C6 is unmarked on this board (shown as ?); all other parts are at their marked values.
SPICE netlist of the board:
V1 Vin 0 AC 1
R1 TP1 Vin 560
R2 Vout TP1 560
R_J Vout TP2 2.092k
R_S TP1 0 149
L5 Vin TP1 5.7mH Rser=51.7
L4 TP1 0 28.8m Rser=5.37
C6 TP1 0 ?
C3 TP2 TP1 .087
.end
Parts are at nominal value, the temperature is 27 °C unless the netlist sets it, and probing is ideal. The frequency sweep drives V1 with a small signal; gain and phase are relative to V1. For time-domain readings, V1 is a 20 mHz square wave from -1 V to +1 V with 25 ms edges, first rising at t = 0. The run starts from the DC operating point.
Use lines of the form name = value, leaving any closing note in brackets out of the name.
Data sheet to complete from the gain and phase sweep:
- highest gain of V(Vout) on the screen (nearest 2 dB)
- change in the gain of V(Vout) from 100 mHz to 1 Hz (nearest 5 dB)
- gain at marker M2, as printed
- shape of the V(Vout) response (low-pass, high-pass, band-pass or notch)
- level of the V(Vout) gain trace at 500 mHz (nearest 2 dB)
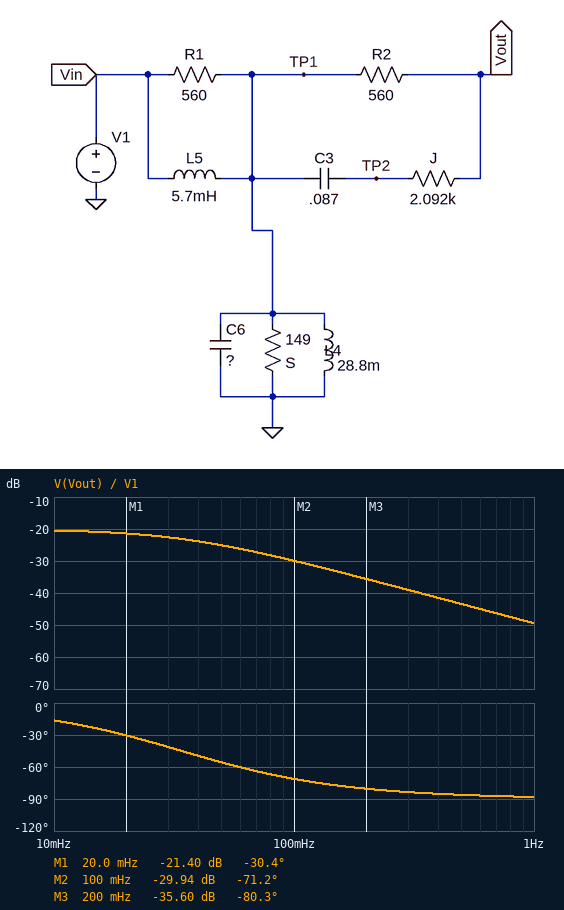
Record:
highest gain of V(Vout) on the screen = -20 dB
change in the gain of V(Vout) from 100 mHz to 1 Hz = -20 dB
gain at marker M2, as printed = -29.94 dB
shape of the V(Vout) response = low-pass
level of the V(Vout) gain trace at 500 mHz = -44 dB
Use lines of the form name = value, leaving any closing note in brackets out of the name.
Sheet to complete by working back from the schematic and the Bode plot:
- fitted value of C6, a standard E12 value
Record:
fitted value of C6, a standard E12 value = 1 F
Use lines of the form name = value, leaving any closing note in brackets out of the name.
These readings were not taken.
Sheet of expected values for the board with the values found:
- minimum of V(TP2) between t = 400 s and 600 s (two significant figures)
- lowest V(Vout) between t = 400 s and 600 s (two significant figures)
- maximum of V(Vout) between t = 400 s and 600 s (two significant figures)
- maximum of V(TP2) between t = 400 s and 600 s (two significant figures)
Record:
minimum of V(TP2) between t = 400 s and 600 s = -98 mV
lowest V(Vout) between t = 400 s and 600 s = -98 mV
maximum of V(Vout) between t = 400 s and 600 s = 98 mV
maximum of V(TP2) between t = 400 s and 600 s = 98 mV
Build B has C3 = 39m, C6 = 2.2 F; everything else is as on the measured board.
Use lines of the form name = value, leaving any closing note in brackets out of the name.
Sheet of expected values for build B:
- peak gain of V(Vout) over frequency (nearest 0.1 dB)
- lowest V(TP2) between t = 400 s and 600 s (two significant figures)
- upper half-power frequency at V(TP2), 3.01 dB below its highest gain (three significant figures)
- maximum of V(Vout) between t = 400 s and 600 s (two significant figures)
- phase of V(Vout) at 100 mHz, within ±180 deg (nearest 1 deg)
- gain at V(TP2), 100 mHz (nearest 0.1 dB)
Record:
peak gain of V(Vout) over frequency = -20.1 dB
lowest V(TP2) between t = 400 s and 600 s = -83 mV
upper half-power frequency at V(TP2), 3.01 dB below its highest gain = 15.5 mHz
maximum of V(Vout) between t = 400 s and 600 s = 83 mV
phase of V(Vout) at 100 mHz, within ±180 deg = -81 deg
gain at V(TP2), 100 mHz = -36.4 dB
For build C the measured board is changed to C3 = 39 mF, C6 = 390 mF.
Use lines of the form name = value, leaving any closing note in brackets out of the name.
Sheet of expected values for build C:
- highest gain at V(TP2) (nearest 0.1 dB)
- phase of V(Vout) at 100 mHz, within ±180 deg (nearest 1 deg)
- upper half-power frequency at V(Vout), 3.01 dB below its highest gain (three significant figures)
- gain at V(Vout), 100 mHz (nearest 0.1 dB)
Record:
highest gain at V(TP2) = -20.1 dB
phase of V(Vout) at 100 mHz, within ±180 deg = -49 deg
upper half-power frequency at V(Vout), 3.01 dB below its highest gain = 87.6 mHz
gain at V(Vout), 100 mHz = -23.7 dB
